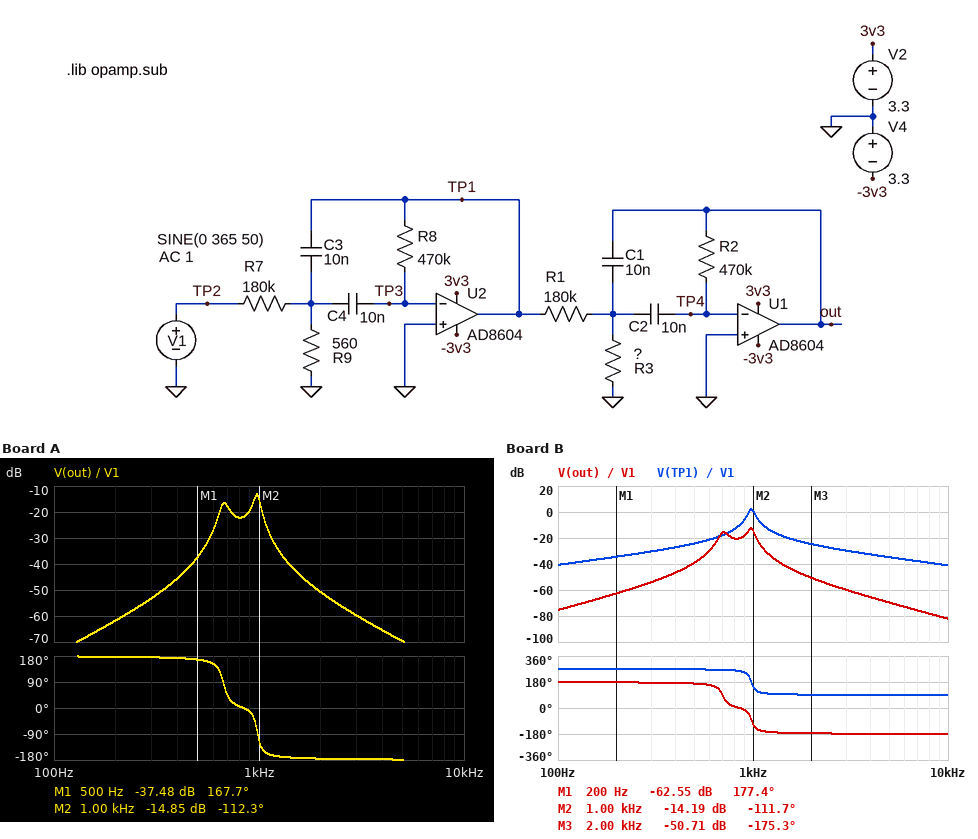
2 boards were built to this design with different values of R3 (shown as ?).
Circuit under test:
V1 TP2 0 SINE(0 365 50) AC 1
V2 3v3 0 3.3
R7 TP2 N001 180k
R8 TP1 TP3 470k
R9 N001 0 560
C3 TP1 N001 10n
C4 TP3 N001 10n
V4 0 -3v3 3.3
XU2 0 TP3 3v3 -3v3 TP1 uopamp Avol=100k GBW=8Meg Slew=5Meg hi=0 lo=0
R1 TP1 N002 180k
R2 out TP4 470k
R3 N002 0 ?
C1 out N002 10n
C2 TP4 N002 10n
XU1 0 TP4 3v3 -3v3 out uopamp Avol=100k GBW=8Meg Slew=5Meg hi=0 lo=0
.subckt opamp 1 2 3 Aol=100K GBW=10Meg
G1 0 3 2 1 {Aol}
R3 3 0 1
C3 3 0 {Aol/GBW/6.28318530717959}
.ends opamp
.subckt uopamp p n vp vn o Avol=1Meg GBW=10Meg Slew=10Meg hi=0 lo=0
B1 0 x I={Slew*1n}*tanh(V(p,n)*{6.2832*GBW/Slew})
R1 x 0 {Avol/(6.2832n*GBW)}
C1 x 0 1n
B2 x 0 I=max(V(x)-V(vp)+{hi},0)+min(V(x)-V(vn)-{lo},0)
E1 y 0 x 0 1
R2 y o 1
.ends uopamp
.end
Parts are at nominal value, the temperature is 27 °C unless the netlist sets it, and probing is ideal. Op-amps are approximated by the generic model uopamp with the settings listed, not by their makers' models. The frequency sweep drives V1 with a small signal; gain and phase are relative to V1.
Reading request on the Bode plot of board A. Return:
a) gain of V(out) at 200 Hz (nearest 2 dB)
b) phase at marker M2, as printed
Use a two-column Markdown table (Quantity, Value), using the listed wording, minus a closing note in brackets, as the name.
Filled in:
| Quantity | Value |
|---|---|
| gain of V(out) at 200 Hz | -62 dB |
| phase at marker M2, as printed | -112.3 deg |
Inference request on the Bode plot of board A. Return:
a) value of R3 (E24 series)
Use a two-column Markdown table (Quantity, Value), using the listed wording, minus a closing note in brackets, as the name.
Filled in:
| Quantity | Value |
|---|---|
| value of R3 | 1.2 kΩ |
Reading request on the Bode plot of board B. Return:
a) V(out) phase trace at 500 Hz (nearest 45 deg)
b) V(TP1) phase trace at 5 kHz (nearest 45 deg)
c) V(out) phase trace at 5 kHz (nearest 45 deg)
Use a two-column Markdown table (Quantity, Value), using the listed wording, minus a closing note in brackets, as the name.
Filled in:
| Quantity | Value |
|---|---|
| V(out) phase trace at 500 Hz | 180 deg |
| V(TP1) phase trace at 5 kHz | 90 deg |
| V(out) phase trace at 5 kHz | -180 deg |
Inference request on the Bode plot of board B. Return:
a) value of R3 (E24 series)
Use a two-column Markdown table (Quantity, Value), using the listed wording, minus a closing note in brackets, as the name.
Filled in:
| Quantity | Value |
|---|---|
| value of R3 | 1.1 kΩ |
